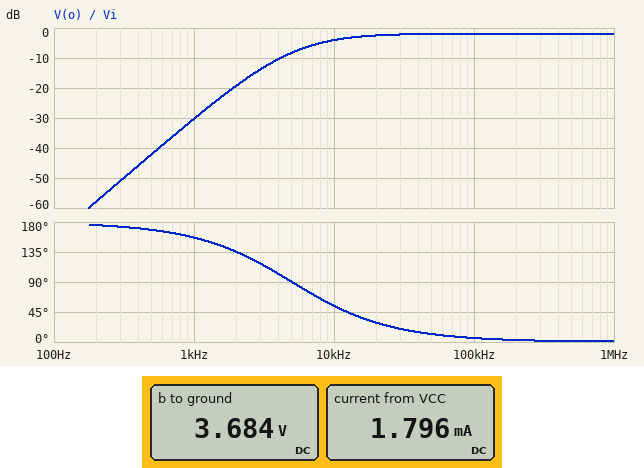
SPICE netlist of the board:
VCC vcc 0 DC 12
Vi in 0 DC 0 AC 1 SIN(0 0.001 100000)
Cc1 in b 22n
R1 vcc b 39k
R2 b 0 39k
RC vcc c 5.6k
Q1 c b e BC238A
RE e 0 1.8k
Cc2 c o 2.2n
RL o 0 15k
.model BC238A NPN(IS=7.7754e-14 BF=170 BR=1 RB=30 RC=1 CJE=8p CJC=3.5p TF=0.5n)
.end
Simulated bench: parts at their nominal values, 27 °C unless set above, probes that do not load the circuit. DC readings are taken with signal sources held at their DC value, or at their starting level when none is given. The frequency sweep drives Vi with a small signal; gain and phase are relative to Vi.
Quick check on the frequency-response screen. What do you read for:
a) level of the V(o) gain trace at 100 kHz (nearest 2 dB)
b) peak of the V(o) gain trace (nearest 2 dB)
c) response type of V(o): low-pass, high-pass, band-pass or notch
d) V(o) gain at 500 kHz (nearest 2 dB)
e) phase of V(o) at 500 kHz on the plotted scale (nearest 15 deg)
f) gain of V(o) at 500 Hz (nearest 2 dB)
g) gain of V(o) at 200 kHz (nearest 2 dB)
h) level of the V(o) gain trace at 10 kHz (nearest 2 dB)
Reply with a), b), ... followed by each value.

a) -2 dB
b) -2 dB
c) high-pass
d) -2 dB
e) 0 deg
f) -42 dB
g) -2 dB
h) -4 dB
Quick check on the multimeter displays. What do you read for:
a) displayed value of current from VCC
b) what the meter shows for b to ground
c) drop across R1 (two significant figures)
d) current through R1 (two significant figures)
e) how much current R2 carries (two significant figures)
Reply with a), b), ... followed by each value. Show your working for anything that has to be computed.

a) 1.796 mA
b) 3.684 V
c) 12 V - 3.684 V = 8.3 V
d) (12 V - 3.684 V) / 39 kΩ = 210 µA
e) (3.684 V) / 39 kΩ = 94 µA
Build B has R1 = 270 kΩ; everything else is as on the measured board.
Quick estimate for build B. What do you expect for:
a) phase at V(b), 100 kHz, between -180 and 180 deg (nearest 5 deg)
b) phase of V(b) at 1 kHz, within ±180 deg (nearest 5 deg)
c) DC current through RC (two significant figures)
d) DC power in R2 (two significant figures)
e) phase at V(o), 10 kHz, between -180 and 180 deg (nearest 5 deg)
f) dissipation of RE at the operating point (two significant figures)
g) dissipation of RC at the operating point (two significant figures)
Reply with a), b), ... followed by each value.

a) 0 deg
b) 15 deg
c) 460 µA
d) 52 µW
e) -160 deg
f) 390 µW
g) 1.2 mW
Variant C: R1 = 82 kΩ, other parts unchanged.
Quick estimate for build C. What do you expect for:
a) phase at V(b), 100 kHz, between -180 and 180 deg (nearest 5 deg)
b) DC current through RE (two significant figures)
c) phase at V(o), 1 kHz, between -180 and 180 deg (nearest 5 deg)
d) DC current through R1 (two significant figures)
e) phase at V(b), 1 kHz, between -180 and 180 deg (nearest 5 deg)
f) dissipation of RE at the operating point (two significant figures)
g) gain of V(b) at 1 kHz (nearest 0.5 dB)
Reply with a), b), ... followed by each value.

a) 0 deg
b) 1.6 mA
c) -35 deg
d) 100 µA
e) 70 deg
f) 4.7 mW
g) -9.0 dB
